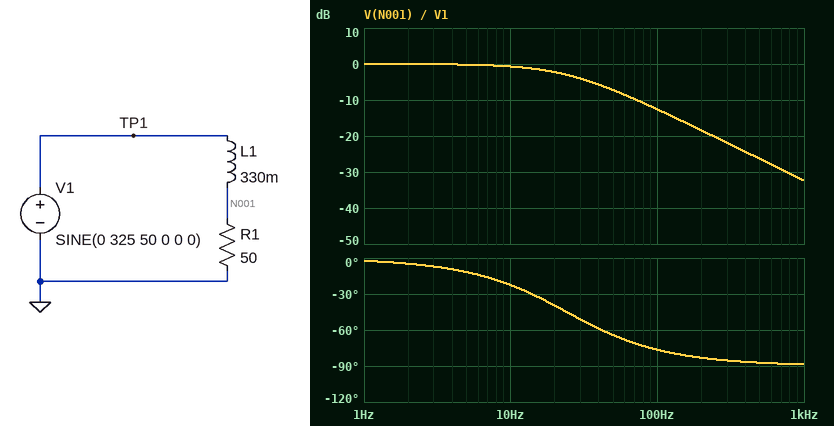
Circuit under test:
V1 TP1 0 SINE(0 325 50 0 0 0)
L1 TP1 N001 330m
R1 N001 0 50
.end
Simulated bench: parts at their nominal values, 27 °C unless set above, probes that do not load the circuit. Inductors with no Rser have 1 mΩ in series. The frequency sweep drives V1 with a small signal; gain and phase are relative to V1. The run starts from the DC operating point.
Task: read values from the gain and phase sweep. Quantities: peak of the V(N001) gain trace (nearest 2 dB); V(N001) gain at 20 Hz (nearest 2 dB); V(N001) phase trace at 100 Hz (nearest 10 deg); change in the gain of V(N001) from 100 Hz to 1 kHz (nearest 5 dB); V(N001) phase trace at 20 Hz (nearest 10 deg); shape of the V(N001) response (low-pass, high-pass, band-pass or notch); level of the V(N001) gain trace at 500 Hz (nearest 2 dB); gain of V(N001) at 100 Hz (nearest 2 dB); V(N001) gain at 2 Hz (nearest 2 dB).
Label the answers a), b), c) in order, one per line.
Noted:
a) 0 dB
b) -2 dB
c) -80 deg
d) -20 dB
e) -40 deg
f) low-pass
g) -26 dB
h) -12 dB
i) 0 dB
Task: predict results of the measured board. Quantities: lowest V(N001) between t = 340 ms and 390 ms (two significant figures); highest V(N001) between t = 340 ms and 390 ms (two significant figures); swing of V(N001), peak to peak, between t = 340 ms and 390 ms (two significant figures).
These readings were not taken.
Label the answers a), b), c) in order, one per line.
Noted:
a) -140 V
b) 140 V
c) 280 V
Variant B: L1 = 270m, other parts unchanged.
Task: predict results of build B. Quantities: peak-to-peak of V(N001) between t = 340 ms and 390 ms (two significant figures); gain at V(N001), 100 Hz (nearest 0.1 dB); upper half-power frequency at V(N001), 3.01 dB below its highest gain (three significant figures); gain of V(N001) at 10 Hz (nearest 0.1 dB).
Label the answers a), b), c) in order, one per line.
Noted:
a) 330 V
b) -11.0 dB
c) 29.5 Hz
d) -0.5 dB
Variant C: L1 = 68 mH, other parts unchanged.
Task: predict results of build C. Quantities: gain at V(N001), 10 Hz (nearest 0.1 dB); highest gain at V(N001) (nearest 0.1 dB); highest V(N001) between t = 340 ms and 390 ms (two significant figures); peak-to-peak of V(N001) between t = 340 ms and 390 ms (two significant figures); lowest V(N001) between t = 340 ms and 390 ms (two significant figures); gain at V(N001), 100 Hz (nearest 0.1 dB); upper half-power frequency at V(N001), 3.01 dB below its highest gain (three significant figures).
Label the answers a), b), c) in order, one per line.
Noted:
a) 0 dB
b) 0 dB
c) 300 V
d) 600 V
e) -300 V
f) -2.4 dB
g) 117 Hz
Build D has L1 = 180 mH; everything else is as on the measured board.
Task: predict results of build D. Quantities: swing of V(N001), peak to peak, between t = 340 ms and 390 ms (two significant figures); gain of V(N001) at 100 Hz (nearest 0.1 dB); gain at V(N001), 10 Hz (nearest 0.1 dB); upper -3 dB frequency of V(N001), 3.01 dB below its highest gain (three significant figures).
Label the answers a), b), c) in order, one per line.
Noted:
a) 430 V
b) -7.9 dB
c) -0.2 dB
d) 44.2 Hz
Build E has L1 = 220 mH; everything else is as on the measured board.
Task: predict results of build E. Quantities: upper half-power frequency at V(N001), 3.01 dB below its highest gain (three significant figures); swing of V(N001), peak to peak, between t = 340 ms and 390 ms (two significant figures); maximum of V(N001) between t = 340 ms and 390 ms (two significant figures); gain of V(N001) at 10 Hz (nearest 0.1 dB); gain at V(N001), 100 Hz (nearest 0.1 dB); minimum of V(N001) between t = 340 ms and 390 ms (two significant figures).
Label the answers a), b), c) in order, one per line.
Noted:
a) 36.2 Hz
b) 380 V
c) 190 V
d) -0.3 dB
e) -9.4 dB
f) -190 V
